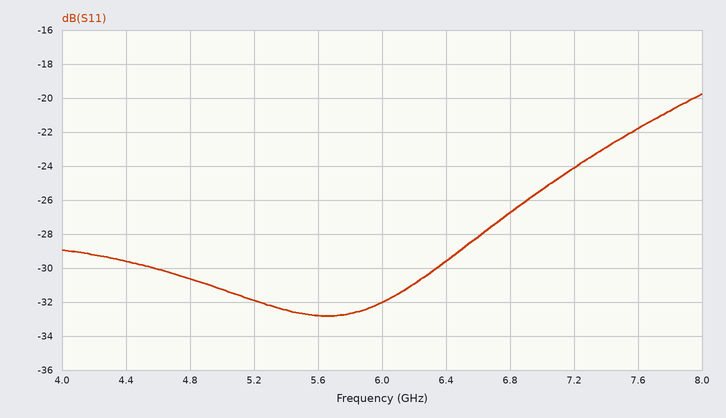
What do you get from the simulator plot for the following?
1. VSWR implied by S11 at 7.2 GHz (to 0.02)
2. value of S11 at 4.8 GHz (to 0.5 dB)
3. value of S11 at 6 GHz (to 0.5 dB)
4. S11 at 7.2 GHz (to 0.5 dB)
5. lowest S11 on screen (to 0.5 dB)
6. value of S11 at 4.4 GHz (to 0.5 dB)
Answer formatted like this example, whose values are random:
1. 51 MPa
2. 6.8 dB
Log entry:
1. 1.14
2. -30.5 dB
3. -32.0 dB
4. -24.0 dB
5. -33.0 dB
6. -29.5 dB
